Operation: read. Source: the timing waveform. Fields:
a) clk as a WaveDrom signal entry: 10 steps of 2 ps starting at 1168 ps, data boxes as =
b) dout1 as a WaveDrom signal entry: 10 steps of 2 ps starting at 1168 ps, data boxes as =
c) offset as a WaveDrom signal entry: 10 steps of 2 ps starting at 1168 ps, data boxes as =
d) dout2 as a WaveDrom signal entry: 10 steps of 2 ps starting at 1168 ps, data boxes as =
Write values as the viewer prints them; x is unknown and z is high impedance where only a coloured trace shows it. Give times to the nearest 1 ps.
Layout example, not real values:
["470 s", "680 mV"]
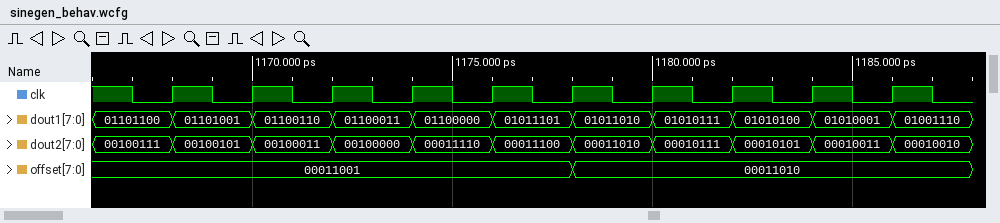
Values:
["{name: 'clk', wave: 'p.........'}", "{name: 'dout1', wave: '==========', data: '01101001 01100110 01100011 01100000 01011101 01011010 01010111 01010100 01010001 01001110'}", "{name: 'offset', wave: '=....=....', data: '00011001 00011010'}", "{name: 'dout2', wave: '==========', data: '00100101 00100011 00100000 00011110 00011100 00011010 00010111 00010101 00010011 00010010'}"]
